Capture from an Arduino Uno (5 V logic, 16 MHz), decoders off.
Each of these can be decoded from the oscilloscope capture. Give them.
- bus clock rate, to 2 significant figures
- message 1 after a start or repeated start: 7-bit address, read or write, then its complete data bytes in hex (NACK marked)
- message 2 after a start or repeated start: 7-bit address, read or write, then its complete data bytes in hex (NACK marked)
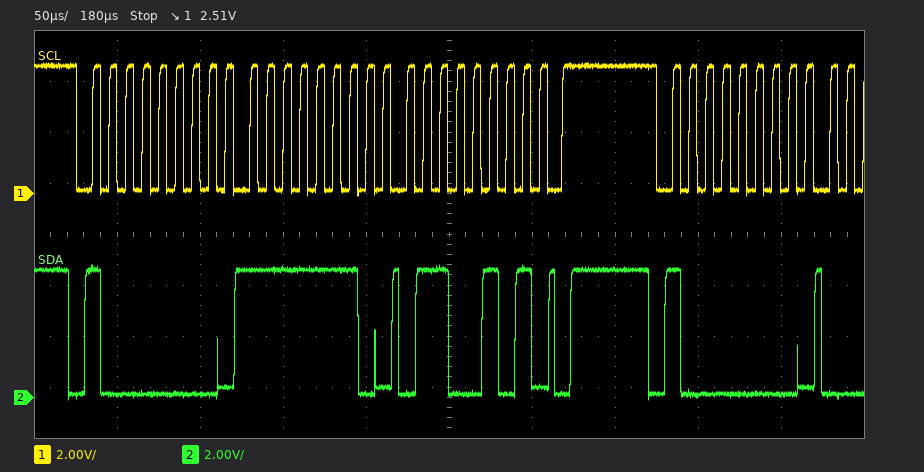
100 kHz
0x40 write: FE 65
0x40 write
